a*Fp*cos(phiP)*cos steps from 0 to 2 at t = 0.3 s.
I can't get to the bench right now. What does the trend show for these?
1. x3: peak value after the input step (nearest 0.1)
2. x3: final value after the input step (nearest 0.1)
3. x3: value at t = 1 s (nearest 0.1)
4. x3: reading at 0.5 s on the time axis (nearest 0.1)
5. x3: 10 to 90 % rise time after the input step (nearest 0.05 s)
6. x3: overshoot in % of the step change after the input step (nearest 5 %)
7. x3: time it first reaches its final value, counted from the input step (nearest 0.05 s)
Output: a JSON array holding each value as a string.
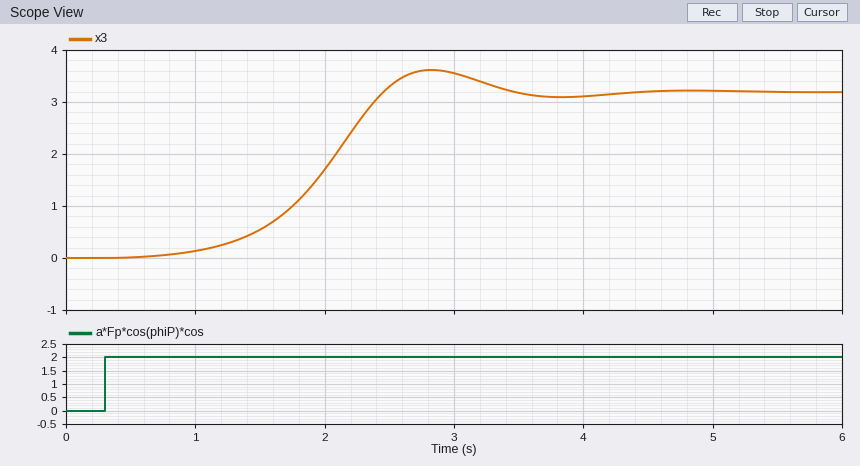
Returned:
["3.6", "3.2", "0.1", "0.0", "1.05 s", "15 %", "2.15 s"]
